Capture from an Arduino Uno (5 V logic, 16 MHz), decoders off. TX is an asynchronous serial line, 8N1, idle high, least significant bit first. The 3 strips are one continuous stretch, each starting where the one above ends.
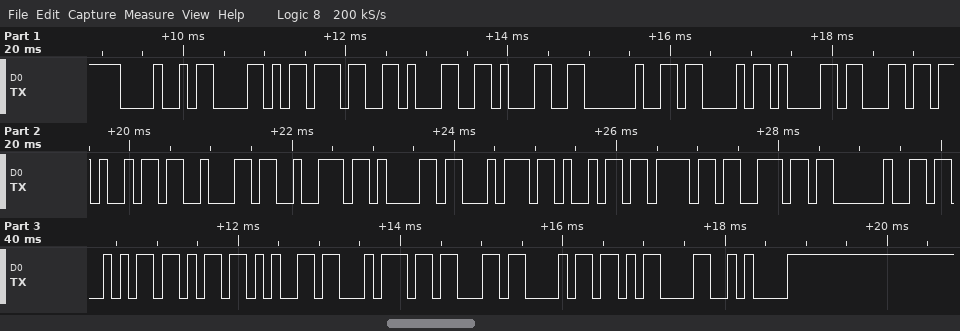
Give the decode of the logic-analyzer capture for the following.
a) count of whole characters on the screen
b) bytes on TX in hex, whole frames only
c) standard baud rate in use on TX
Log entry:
26
48 58 37 31 31 20 43 61 6C 69 62 72 61 74 69 6F 6E 20 53 6B 65 74 63 68 0D 0A
9600 baud
